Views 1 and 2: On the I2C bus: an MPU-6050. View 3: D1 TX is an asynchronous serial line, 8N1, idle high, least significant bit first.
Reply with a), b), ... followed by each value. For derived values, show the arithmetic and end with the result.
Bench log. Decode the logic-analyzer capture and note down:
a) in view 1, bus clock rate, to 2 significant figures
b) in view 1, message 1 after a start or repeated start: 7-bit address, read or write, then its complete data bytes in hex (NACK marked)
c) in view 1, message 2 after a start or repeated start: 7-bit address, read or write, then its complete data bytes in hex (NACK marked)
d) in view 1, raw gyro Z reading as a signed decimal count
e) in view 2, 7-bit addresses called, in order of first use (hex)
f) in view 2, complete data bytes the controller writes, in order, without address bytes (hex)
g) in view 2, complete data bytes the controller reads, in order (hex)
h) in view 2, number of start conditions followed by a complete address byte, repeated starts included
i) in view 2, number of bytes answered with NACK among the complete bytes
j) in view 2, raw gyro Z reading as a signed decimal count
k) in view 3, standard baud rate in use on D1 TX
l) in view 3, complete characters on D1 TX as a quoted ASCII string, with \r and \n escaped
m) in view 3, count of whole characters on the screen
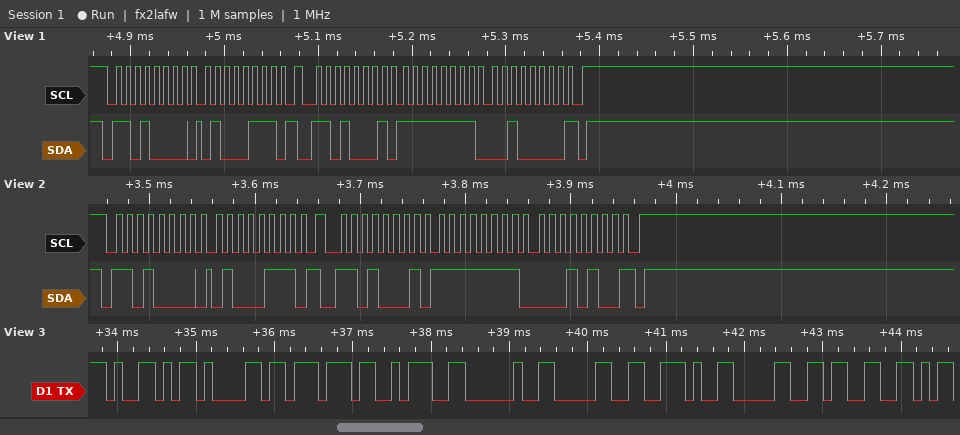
a) 100 kHz
b) 0x68 write: 47
c) 0x68 read: FF 20 NACK
d) 0xFF20 = -224
e) 0x68
f) 47
g) FF 14
h) 2
i) 1
j) 0xFF14 = -236
k) 9600 baud
l) "Yaw: 0.03"
m) 9
